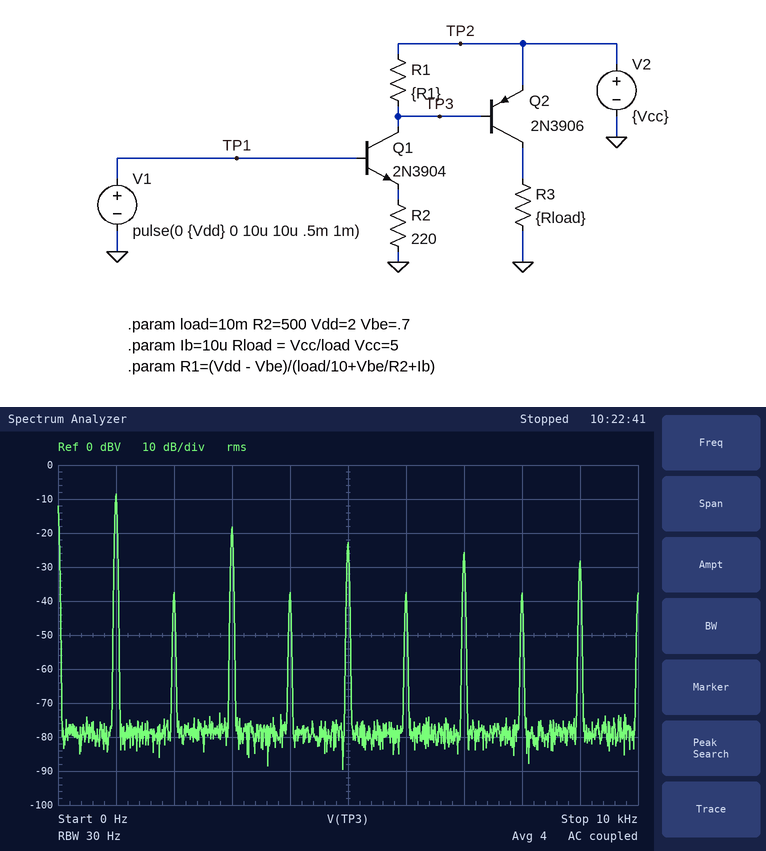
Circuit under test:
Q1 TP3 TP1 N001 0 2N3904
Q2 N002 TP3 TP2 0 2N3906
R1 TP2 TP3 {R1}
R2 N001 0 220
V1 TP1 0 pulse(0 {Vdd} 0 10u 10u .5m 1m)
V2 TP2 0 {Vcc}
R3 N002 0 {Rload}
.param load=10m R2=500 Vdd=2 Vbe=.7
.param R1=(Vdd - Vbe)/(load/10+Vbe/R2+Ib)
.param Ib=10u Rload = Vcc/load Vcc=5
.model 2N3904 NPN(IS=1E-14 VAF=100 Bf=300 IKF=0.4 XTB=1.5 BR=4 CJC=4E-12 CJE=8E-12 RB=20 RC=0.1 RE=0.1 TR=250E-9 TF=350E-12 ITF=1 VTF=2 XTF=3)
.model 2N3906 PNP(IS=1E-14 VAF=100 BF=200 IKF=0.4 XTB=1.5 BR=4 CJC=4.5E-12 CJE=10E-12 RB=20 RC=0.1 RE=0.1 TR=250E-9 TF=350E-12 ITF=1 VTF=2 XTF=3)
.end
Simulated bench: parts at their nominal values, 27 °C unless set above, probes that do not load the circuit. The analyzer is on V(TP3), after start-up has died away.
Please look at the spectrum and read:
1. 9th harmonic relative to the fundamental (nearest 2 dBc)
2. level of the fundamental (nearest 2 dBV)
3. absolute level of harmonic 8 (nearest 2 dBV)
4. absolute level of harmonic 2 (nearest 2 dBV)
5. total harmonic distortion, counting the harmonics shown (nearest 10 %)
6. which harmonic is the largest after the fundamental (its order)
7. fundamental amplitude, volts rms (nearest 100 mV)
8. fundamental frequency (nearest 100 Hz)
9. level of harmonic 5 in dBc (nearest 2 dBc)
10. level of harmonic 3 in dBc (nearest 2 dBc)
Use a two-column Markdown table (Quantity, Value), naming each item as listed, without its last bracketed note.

| Quantity | Value |
|---|---|
| 9th harmonic relative to the fundamental | -20 dBc |
| level of the fundamental | -8 dBV |
| absolute level of harmonic 8 | -38 dBV |
| absolute level of harmonic 2 | -38 dBV |
| total harmonic distortion, counting the harmonics shown | 40 % |
| which harmonic is the largest after the fundamental | 3 |
| fundamental amplitude, volts rms | 400 mV |
| fundamental frequency | 1.0 kHz |
| level of harmonic 5 in dBc | -14 dBc |
| level of harmonic 3 in dBc | -10 dBc |
